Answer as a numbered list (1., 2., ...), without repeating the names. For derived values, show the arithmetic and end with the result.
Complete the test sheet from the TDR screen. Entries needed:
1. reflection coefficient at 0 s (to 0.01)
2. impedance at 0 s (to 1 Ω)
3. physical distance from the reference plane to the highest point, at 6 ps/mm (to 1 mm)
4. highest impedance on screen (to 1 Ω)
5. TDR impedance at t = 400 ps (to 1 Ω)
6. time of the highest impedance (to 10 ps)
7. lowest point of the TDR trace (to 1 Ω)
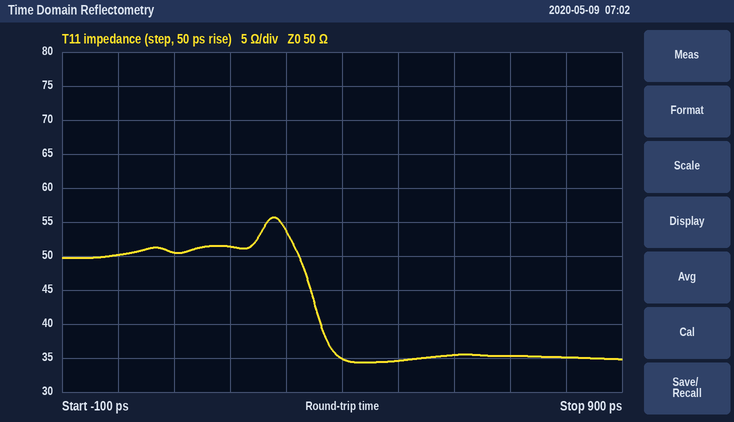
1. (50 − 50)/(50 + 50) ≈ 0.00
2. 50 Ω
3. 280 ps / 2 / 6 ps/mm ≈ 23 mm
4. 56 Ω
5. 35 Ω
6. 280 ps
7. 34 Ω
